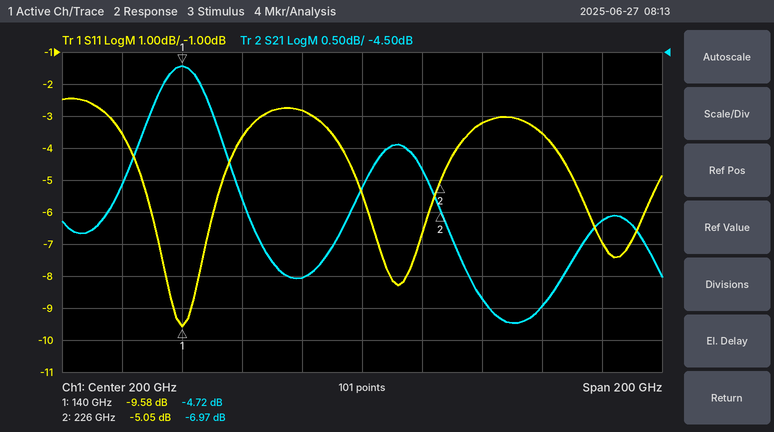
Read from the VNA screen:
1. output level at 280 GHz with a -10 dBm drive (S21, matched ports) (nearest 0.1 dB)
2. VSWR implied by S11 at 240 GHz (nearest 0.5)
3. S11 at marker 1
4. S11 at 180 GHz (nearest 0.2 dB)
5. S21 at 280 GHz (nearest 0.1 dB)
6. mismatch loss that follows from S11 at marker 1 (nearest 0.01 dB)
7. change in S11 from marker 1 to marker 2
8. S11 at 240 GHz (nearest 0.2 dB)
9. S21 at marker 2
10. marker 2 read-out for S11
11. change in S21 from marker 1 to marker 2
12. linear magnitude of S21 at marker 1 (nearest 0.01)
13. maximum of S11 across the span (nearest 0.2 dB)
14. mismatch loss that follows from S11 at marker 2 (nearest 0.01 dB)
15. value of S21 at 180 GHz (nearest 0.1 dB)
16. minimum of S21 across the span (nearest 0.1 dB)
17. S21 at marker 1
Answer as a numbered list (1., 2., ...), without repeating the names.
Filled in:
1. -17.1 dBm
2. 5.5
3. -9.58 dB
4. -2.8 dB
5. -7.1 dB
6. 0.51 dB
7. 4.53 dB
8. -3.2 dB
9. -6.97 dB
10. -5.05 dB
11. -2.25 dB
12. 0.58
13. -2.4 dB
14. 1.63 dB
15. -8.0 dB
16. -8.7 dB
17. -4.72 dB
